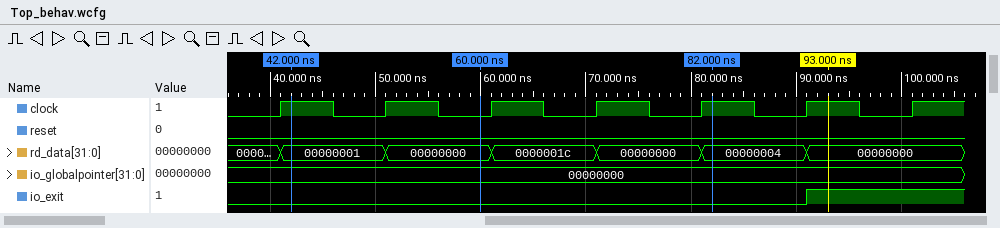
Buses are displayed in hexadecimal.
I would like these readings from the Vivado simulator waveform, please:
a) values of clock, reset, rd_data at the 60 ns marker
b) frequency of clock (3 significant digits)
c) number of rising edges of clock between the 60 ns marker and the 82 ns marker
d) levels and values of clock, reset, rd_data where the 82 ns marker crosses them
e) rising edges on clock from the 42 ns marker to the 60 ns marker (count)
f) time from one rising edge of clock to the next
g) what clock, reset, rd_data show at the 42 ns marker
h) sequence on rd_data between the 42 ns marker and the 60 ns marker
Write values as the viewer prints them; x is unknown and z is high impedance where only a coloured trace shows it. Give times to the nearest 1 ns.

clock=0, reset=0, rd_data=00000000
100 MHz
3
clock=1, reset=0, rd_data=00000004
1
10 ns
clock=1, reset=0, rd_data=00000001
00000001, 00000000
